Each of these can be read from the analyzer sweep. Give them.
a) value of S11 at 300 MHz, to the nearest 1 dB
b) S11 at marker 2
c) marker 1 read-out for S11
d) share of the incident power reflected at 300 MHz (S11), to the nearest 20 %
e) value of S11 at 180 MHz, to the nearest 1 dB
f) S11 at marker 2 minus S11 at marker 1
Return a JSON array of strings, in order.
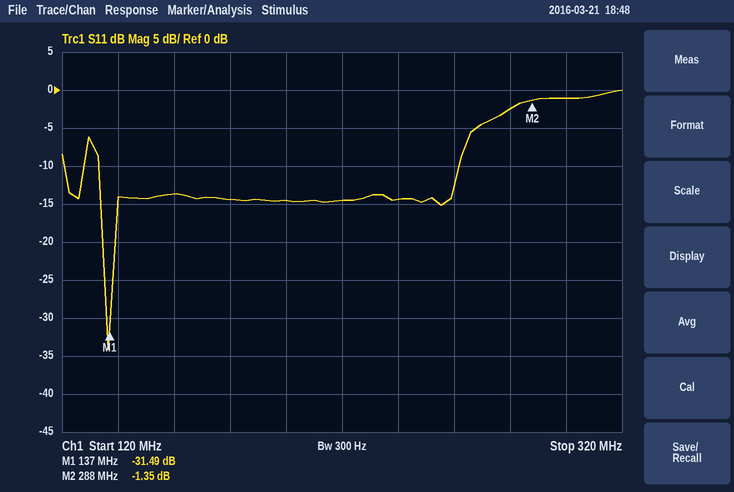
["-1 dB", "-1.35 dB", "-31.49 dB", "80 %", "-14 dB", "30.14 dB"]
